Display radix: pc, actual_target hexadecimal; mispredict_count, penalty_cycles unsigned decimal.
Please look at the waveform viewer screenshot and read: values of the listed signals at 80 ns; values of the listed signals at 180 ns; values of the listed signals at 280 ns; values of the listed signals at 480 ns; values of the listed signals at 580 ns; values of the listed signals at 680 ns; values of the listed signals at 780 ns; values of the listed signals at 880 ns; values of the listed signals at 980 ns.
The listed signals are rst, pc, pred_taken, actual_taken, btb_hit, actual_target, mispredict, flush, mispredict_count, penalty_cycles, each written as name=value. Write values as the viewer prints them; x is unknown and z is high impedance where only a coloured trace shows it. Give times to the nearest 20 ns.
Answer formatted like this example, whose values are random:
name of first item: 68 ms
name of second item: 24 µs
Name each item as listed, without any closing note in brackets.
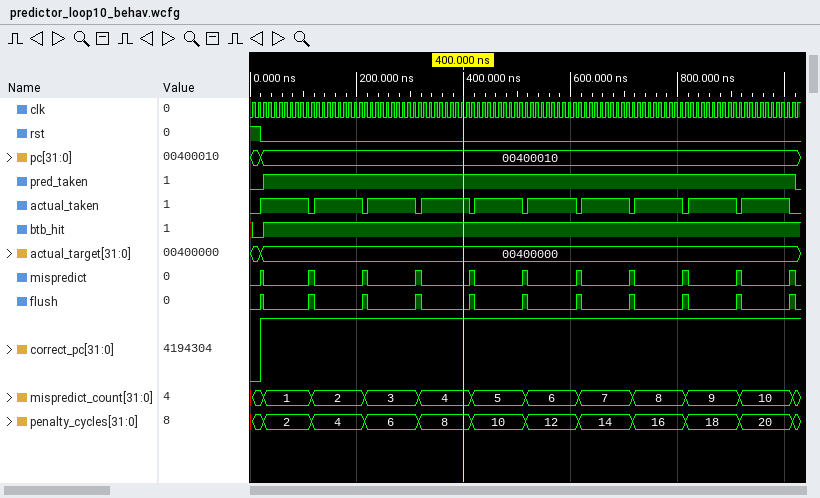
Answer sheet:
values of the listed signals at 80 ns: rst=0, pc=00400010, pred_taken=1, actual_taken=1, btb_hit=1, actual_target=00400000, mispredict=0, flush=0, mispredict_count=1, penalty_cycles=2
values of the listed signals at 180 ns: rst=0, pc=00400010, pred_taken=1, actual_taken=1, btb_hit=1, actual_target=00400000, mispredict=0, flush=0, mispredict_count=2, penalty_cycles=4
values of the listed signals at 280 ns: rst=0, pc=00400010, pred_taken=1, actual_taken=1, btb_hit=1, actual_target=00400000, mispredict=0, flush=0, mispredict_count=3, penalty_cycles=6
values of the listed signals at 480 ns: rst=0, pc=00400010, pred_taken=1, actual_taken=1, btb_hit=1, actual_target=00400000, mispredict=0, flush=0, mispredict_count=5, penalty_cycles=10
values of the listed signals at 580 ns: rst=0, pc=00400010, pred_taken=1, actual_taken=1, btb_hit=1, actual_target=00400000, mispredict=0, flush=0, mispredict_count=6, penalty_cycles=12
values of the listed signals at 680 ns: rst=0, pc=00400010, pred_taken=1, actual_taken=1, btb_hit=1, actual_target=00400000, mispredict=0, flush=0, mispredict_count=7, penalty_cycles=14
values of the listed signals at 780 ns: rst=0, pc=00400010, pred_taken=1, actual_taken=1, btb_hit=1, actual_target=00400000, mispredict=0, flush=0, mispredict_count=8, penalty_cycles=16
values of the listed signals at 880 ns: rst=0, pc=00400010, pred_taken=1, actual_taken=1, btb_hit=1, actual_target=00400000, mispredict=0, flush=0, mispredict_count=9, penalty_cycles=18
values of the listed signals at 980 ns: rst=0, pc=00400010, pred_taken=1, actual_taken=1, btb_hit=1, actual_target=00400000, mispredict=0, flush=0, mispredict_count=10, penalty_cycles=20
